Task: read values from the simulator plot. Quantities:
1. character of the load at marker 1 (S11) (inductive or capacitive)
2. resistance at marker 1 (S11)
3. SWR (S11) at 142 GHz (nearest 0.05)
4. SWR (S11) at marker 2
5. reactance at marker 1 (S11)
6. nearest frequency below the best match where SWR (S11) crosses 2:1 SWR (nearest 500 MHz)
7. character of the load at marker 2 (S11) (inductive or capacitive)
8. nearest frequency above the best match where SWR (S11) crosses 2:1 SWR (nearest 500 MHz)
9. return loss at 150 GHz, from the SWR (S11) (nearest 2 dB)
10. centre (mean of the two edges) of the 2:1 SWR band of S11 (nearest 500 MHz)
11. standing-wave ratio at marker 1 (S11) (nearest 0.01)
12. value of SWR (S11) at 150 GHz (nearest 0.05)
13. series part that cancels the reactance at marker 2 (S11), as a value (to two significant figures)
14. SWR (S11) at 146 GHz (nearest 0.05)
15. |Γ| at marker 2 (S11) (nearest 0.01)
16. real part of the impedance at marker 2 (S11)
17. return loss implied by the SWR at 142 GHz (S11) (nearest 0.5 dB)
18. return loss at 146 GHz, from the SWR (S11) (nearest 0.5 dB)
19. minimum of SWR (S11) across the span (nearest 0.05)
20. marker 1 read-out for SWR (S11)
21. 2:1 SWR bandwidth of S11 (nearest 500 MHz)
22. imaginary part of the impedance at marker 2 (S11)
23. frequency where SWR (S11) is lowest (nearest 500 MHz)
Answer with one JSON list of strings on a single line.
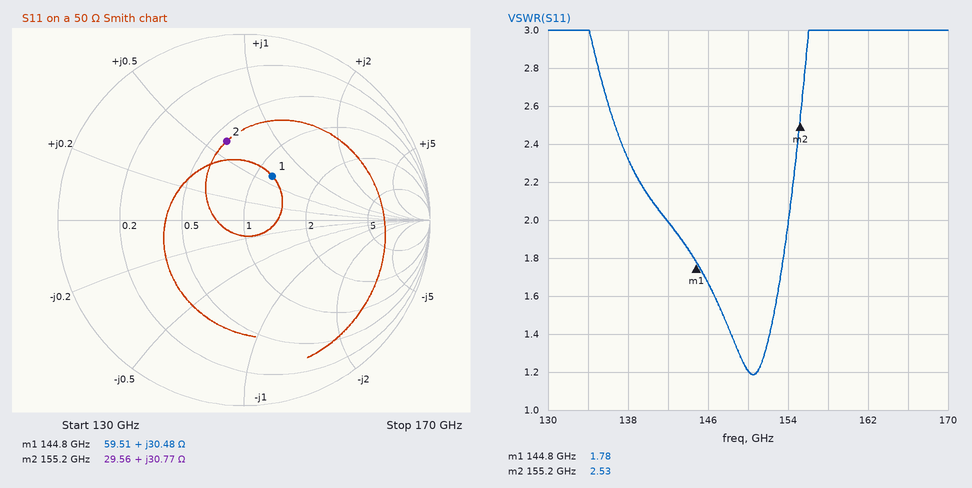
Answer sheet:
["inductive", "59.51 Ω", "2.00", "2.53", "+30.48 Ω", "142.0 GHz", "inductive", "154.0 GHz", "20 dB", "148.0 GHz", "1.78", "1.20", "33 fF", "1.65", "0.43", "29.56 Ω", "9.5 dB", "12.0 dB", "1.20", "1.78", "12.0 GHz", "+30.77 Ω", "150.5 GHz"]
